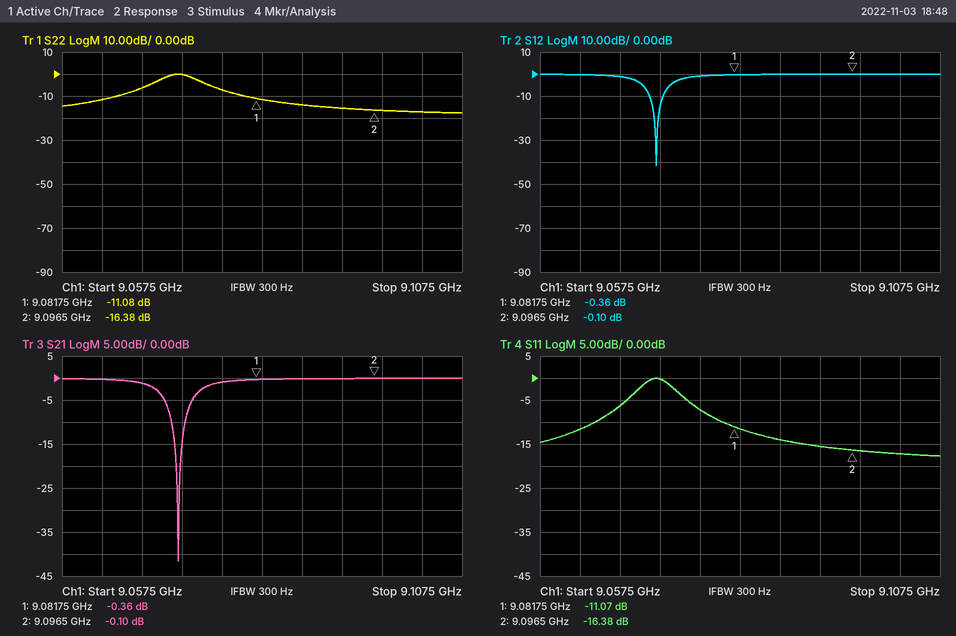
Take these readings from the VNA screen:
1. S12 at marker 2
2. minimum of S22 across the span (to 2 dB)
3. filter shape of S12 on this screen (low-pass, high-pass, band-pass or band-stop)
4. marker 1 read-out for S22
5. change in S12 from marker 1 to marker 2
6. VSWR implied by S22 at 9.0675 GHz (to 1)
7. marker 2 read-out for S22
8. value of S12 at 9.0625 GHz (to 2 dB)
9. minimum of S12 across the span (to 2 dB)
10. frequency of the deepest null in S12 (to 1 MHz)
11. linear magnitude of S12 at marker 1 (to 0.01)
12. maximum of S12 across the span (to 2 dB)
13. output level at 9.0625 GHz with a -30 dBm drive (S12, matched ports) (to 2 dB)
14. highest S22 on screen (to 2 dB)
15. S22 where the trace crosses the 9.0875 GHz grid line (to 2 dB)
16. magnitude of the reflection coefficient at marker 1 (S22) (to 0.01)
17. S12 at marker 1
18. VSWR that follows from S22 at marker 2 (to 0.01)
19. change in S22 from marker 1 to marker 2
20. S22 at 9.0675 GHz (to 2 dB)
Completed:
-0.10 dB
-18 dB
band-stop
-11.08 dB
0.26 dB
3
-16.38 dB
0 dB
-42 dB
9.072 GHz
0.96
0 dB
-30 dBm
0 dB
-14 dB
0.28
-0.36 dB
1.36
-5.30 dB
-6 dB
